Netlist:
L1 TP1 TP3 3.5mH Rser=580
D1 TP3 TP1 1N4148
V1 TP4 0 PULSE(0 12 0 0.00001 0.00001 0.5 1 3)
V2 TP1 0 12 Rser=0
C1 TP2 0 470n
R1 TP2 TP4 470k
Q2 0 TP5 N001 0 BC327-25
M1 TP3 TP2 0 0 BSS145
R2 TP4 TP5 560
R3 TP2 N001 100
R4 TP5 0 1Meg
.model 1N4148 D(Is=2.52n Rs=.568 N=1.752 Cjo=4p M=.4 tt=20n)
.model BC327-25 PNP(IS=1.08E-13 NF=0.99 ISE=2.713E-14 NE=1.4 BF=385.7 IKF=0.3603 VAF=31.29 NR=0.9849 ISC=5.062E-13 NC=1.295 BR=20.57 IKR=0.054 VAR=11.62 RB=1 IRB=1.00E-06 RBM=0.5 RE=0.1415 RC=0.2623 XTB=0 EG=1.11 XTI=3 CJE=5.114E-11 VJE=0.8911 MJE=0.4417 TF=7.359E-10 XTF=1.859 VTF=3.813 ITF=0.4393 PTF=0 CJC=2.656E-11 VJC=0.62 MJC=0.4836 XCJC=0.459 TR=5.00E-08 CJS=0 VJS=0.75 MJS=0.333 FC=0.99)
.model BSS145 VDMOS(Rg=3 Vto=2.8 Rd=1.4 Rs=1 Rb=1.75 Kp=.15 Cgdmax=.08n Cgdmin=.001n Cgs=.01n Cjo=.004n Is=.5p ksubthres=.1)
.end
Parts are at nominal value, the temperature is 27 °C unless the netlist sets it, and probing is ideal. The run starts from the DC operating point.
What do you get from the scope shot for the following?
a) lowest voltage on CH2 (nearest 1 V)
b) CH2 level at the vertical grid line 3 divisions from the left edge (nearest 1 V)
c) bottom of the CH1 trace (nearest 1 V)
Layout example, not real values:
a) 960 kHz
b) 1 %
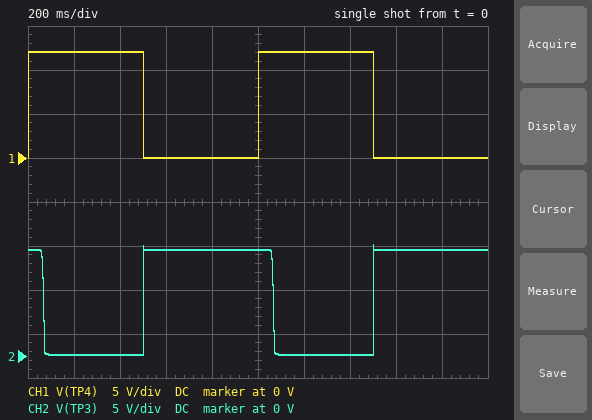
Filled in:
a) 0 V
b) 12 V
c) 0 V
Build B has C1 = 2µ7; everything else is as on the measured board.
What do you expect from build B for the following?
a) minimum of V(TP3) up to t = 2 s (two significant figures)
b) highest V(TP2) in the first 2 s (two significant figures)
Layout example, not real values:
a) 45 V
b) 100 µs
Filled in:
a) 160 mV
b) 4.1 V
